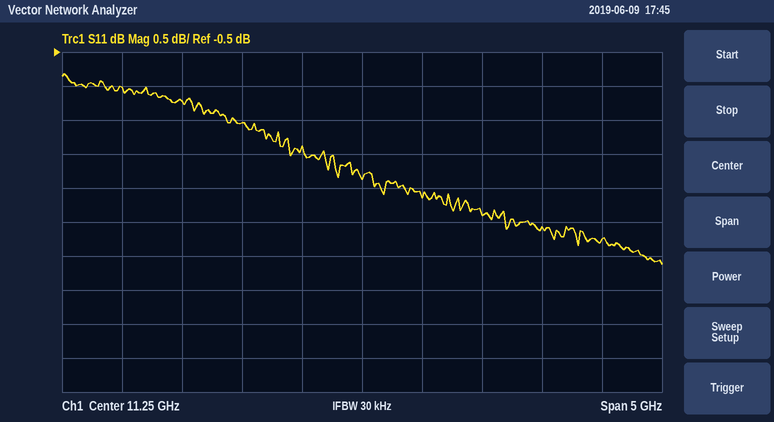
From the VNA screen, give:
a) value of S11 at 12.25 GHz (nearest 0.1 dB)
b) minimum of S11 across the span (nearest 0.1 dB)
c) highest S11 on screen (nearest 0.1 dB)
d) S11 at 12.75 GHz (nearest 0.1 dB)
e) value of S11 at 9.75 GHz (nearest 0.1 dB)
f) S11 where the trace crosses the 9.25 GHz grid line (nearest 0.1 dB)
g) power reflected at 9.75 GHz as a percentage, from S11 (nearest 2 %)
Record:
-2.9 dB
-3.6 dB
-0.8 dB
-3.1 dB
-1.2 dB
-1.0 dB
76 %
